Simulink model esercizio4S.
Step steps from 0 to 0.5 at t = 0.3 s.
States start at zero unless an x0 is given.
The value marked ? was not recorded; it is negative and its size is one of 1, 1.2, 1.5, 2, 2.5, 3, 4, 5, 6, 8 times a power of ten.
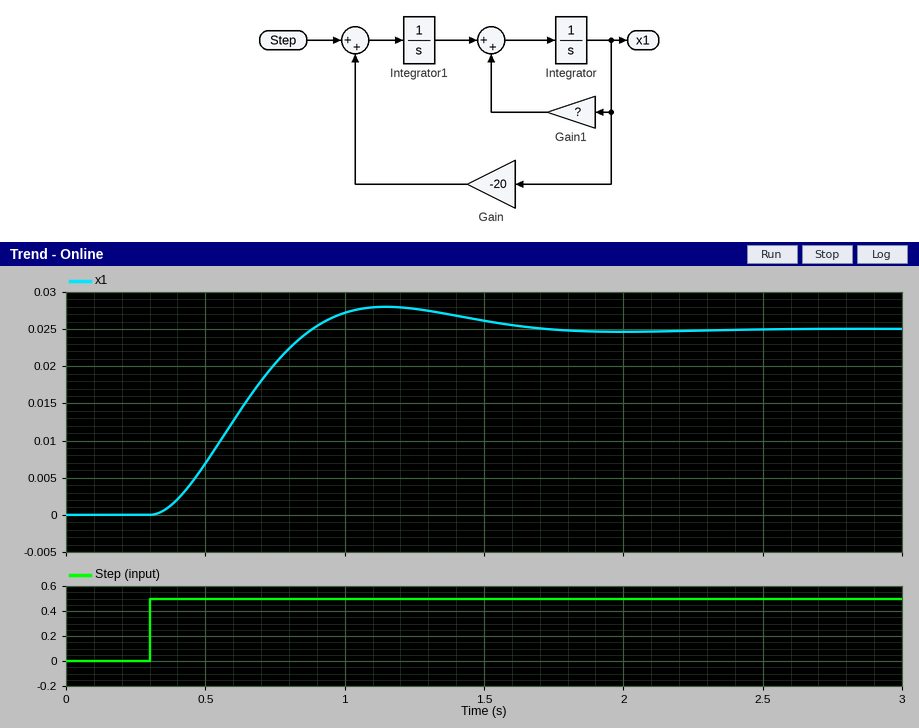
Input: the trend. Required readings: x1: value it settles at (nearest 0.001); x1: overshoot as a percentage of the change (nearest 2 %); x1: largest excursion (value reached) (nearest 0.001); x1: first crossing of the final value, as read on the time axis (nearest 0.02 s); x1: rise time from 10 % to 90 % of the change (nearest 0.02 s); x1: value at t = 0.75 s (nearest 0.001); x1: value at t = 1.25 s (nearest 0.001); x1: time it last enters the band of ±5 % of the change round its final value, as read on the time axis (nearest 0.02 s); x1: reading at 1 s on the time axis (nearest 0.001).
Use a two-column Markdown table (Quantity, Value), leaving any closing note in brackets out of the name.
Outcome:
| Quantity | Value |
|---|---|
| x1: value it settles at | 0.025 |
| x1: overshoot as a percentage of the change | 12 % |
| x1: largest excursion (value reached) | 0.028 |
| x1: first crossing of the final value, as read on the time axis | 0.88 s |
| x1: rise time from 10 % to 90 % of the change | 0.40 s |
| x1: value at t = 0.75 s | 0.020 |
| x1: value at t = 1.25 s | 0.028 |
| x1: time it last enters the band of ±5 % of the change round its final value, as read on the time axis | 1.48 s |
| x1: reading at 1 s on the time axis | 0.027 |
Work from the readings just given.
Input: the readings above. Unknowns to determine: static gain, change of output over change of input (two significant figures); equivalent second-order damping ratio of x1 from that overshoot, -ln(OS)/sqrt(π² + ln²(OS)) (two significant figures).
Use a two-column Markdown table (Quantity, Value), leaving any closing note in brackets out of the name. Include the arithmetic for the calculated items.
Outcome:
| Quantity | Value |
|---|---|
| static gain, change of output over change of input | (0.025 - 0) / (0.5 - 0) = 0.050 |
| equivalent second-order damping ratio of x1 from that overshoot, -ln(OS)/sqrt(π² + ln²(OS)) | ln(0.12) = -2.120; 2.120 / sqrt(9.870 + 4.496) = 0.56 |
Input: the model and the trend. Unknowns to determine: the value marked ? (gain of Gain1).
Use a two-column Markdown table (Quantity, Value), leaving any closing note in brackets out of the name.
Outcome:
| Quantity | Value |
|---|---|
| the value marked ? | -5 |
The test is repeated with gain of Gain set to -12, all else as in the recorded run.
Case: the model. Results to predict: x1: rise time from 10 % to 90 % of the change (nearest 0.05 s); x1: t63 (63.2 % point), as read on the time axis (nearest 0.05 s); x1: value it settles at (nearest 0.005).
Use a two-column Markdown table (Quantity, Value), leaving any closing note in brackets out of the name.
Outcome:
| Quantity | Value |
|---|---|
| x1: rise time from 10 % to 90 % of the change | 0.65 s |
| x1: t63 (63.2 % point), as read on the time axis | 0.80 s |
| x1: value it settles at | 0.040 |
